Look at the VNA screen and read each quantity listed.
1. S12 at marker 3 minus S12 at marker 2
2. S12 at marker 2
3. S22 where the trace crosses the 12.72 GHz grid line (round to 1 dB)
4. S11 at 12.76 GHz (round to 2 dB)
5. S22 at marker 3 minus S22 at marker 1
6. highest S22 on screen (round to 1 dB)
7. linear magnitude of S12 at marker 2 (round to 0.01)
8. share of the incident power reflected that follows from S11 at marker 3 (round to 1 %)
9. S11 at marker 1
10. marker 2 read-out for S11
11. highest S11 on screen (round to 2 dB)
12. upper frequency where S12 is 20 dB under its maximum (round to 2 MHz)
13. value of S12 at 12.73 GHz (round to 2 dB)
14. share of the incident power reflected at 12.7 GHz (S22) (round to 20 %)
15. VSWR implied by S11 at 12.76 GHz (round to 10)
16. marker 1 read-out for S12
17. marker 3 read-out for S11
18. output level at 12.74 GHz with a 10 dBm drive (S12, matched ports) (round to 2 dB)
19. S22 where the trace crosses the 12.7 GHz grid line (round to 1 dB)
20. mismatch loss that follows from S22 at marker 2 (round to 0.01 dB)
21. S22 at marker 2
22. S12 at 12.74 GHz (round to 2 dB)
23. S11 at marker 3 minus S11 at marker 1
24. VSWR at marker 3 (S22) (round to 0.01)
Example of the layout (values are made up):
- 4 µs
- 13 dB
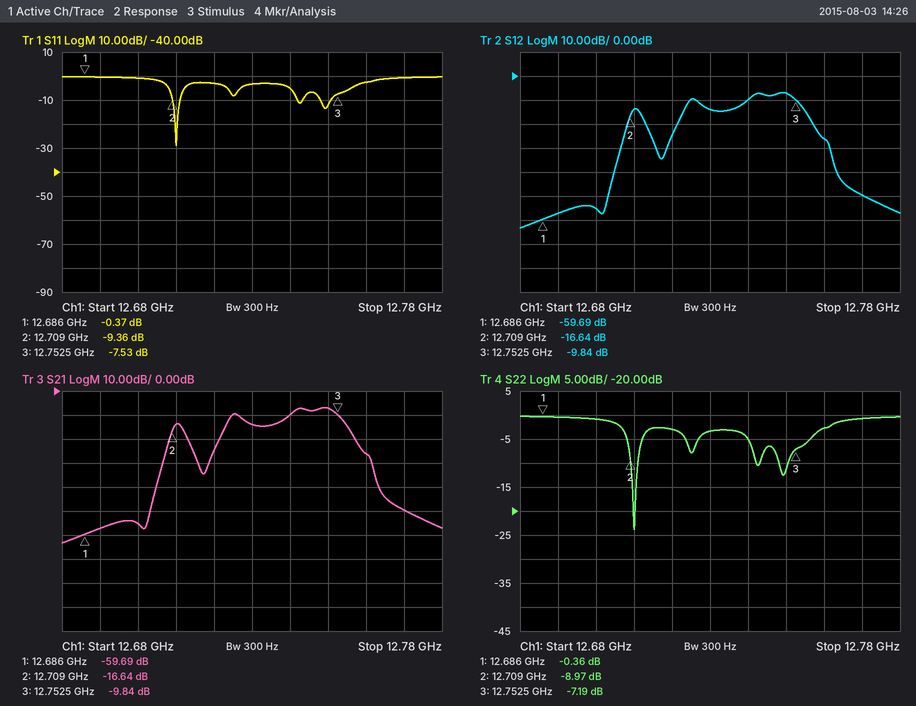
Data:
- 6.80 dB
- -16.64 dB
- -3 dB
- -2 dB
- -6.83 dB
- 0 dB
- 0.15
- 18 %
- -0.37 dB
- -9.36 dB
- 0 dB
- 12.760 GHz
- -14 dB
- 80 %
- 10
- -59.69 dB
- -7.53 dB
- 0 dBm
- -1 dB
- 0.59 dB
- -8.97 dB
- -10 dB
- -7.16 dB
- 2.55
